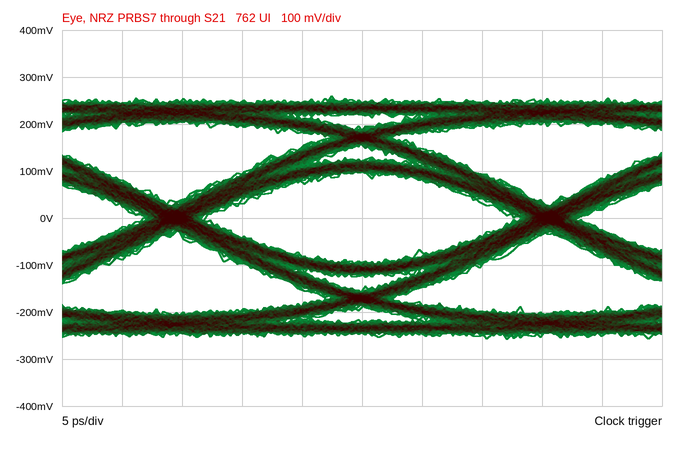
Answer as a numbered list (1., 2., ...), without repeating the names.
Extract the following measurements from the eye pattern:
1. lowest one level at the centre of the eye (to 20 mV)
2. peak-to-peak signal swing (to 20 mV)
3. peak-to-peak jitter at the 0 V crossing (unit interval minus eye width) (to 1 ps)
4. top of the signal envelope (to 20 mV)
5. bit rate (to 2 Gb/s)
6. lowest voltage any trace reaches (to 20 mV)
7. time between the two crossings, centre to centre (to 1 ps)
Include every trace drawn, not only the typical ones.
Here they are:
1. 100 mV
2. 520 mV
3. 5 ps
4. 260 mV
5. 32 Gb/s
6. -260 mV
7. 31 ps
